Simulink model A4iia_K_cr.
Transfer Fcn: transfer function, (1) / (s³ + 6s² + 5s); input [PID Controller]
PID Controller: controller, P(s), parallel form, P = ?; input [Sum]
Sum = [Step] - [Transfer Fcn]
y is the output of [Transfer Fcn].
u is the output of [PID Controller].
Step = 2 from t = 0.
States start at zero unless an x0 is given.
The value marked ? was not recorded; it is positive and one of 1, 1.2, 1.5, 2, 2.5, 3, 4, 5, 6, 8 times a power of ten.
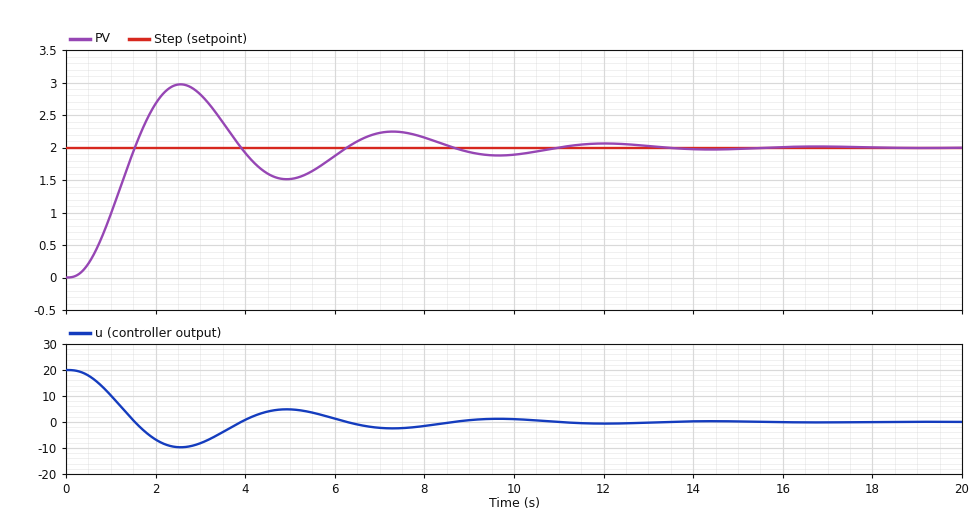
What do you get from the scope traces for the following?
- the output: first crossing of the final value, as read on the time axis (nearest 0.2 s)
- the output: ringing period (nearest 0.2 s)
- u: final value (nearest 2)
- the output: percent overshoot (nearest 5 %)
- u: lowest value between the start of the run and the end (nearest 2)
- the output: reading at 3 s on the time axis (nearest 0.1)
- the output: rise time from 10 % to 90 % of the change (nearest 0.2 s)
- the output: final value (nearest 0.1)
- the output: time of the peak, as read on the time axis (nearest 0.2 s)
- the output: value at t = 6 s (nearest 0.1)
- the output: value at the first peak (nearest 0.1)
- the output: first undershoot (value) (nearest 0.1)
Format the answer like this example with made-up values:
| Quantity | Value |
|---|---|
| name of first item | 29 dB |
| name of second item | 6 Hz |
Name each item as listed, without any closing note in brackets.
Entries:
| Quantity | Value |
|---|---|
| the output: first crossing of the final value, as read on the time axis | 1.6 s |
| the output: ringing period | 4.8 s |
| u: final value | 0 |
| the output: percent overshoot | 50 % |
| u: lowest value between the start of the run and the end | -10 |
| the output: reading at 3 s on the time axis | 2.8 |
| the output: rise time from 10 % to 90 % of the change | 1.0 s |
| the output: final value | 2.0 |
| the output: time of the peak, as read on the time axis | 2.6 s |
| the output: value at t = 6 s | 1.9 |
| the output: value at the first peak | 3.0 |
| the output: first undershoot (value) | 1.5 |
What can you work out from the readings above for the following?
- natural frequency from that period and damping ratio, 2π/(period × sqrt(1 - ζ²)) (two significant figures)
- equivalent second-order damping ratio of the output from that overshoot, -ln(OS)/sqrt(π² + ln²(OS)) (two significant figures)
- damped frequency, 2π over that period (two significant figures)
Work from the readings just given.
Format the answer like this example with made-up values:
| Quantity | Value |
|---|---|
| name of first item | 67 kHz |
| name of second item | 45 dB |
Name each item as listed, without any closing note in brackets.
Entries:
| Quantity | Value |
|---|---|
| natural frequency from that period and damping ratio, 2π/(period × sqrt(1 - ζ²)) | 1.3 rad/s |
| equivalent second-order damping ratio of the output from that overshoot, -ln(OS)/sqrt(π² + ln²(OS)) | 0.22 |
| damped frequency, 2π over that period | 1.3 rad/s |
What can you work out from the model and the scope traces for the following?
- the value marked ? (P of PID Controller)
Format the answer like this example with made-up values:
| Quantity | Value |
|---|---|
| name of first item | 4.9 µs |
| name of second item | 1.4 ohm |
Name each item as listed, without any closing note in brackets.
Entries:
| Quantity | Value |
|---|---|
| the value marked ? | 10 |
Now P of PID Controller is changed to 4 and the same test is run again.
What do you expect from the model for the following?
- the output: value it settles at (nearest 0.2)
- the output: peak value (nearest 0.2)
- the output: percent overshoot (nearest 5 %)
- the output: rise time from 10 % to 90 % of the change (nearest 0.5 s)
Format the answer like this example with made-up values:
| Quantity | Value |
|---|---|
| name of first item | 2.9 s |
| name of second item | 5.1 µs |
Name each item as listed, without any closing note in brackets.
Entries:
| Quantity | Value |
|---|---|
| the output: value it settles at | 2.0 |
| the output: peak value | 2.4 |
| the output: percent overshoot | 20 % |
| the output: rise time from 10 % to 90 % of the change | 2.0 s |
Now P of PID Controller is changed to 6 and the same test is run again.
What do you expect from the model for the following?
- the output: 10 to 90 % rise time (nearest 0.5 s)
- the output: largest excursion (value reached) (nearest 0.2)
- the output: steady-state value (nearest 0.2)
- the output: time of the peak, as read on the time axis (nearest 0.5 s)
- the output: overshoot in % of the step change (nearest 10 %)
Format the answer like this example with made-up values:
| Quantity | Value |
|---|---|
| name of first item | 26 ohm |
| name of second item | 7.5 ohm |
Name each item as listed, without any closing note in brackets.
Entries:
| Quantity | Value |
|---|---|
| the output: 10 to 90 % rise time | 1.5 s |
| the output: largest excursion (value reached) | 2.6 |
| the output: steady-state value | 2.0 |
| the output: time of the peak, as read on the time axis | 3.5 s |
| the output: overshoot in % of the step change | 30 % |
